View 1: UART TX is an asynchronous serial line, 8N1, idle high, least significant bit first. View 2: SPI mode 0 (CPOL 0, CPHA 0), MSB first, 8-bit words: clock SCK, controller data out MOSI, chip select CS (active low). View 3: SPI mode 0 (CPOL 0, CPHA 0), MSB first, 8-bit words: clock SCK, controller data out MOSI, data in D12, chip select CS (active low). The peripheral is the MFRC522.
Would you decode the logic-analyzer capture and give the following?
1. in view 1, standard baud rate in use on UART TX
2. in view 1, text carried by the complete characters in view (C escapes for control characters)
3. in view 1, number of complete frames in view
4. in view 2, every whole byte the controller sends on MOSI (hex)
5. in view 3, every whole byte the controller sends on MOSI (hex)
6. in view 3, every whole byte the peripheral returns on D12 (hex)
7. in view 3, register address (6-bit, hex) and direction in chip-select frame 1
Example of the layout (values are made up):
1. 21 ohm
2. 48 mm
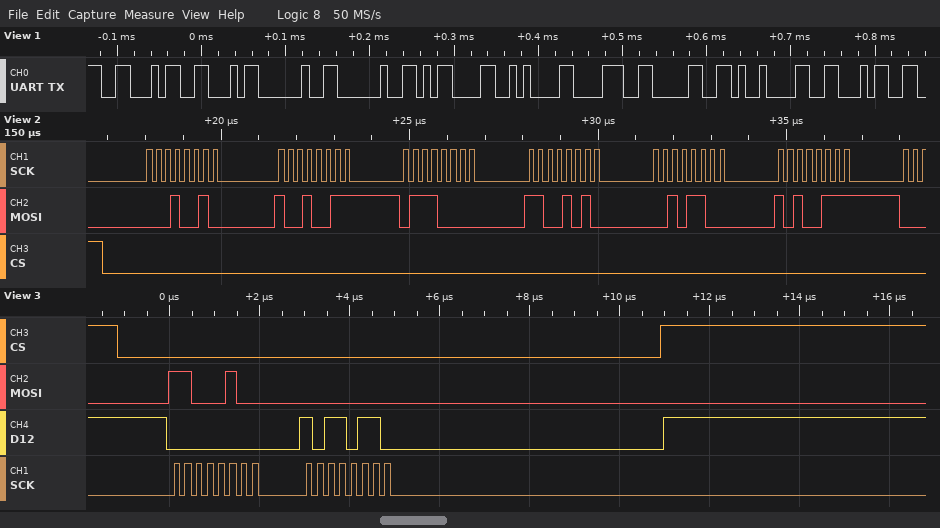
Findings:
1. 115200 baud
2. "FF  \r\n80\tF"
3. 10
4. 0x12 0x93 0x70 0xCA 0x2C 0xA7
5. C4 00
6. 00 B6
7. 0x22 read
